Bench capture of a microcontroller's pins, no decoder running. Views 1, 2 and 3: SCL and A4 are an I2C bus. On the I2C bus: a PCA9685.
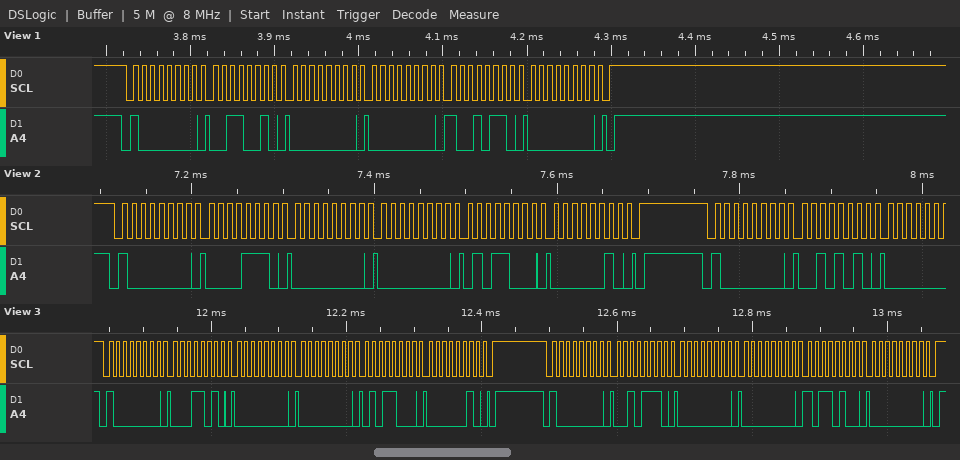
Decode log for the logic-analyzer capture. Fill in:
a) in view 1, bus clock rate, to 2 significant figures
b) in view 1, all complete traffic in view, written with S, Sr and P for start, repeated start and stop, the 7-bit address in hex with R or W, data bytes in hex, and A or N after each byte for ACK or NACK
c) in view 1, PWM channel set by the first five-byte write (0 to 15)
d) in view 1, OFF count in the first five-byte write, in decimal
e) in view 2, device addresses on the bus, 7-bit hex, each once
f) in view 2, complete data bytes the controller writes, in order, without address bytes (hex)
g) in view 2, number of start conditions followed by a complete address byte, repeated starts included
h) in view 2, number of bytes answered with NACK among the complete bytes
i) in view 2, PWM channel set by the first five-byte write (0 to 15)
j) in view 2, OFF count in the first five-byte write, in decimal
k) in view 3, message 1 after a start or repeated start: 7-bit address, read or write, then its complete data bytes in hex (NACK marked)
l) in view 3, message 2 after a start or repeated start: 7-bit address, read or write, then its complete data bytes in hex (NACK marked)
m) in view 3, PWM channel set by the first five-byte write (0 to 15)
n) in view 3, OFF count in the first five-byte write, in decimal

100 kHz
S 40W A 32 A 00 A 00 A 96 A 00 A P
11
150
0x40
0E 00 00 58 02 2A
2
0
2
600
0x40 write: 1A 00 00 58 02
0x40 write: 2E 00 00 B4 00
5
600
